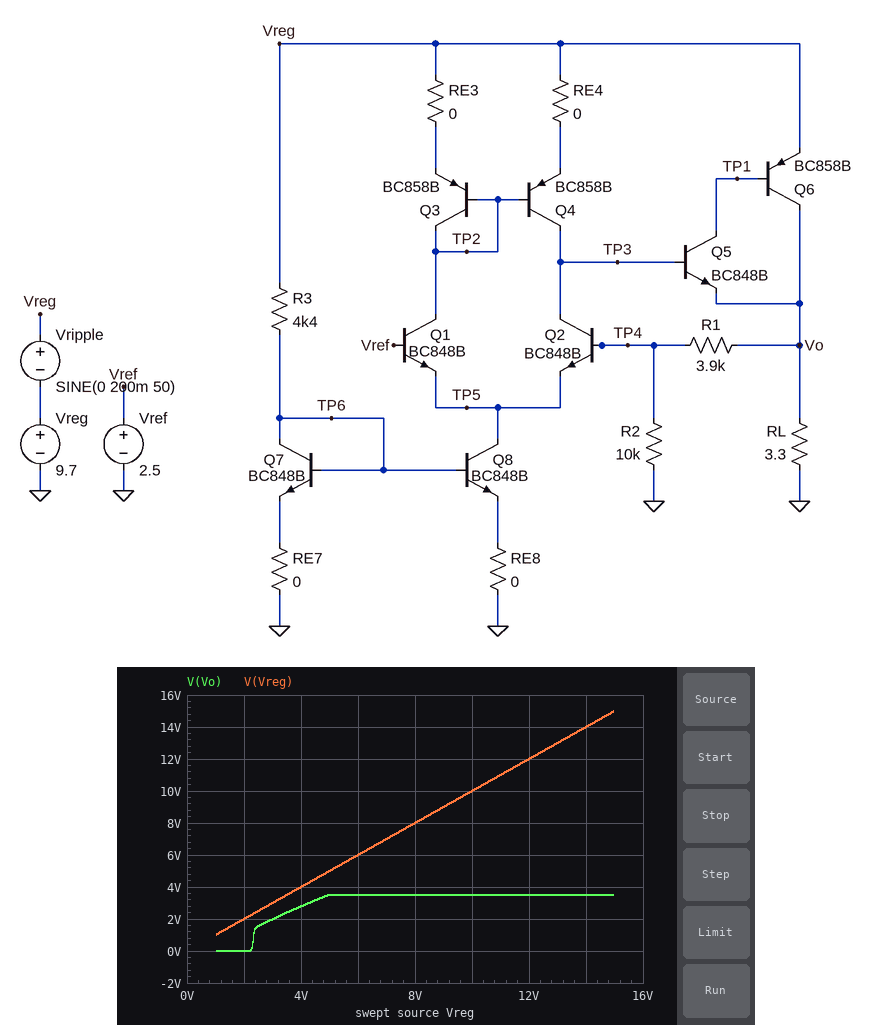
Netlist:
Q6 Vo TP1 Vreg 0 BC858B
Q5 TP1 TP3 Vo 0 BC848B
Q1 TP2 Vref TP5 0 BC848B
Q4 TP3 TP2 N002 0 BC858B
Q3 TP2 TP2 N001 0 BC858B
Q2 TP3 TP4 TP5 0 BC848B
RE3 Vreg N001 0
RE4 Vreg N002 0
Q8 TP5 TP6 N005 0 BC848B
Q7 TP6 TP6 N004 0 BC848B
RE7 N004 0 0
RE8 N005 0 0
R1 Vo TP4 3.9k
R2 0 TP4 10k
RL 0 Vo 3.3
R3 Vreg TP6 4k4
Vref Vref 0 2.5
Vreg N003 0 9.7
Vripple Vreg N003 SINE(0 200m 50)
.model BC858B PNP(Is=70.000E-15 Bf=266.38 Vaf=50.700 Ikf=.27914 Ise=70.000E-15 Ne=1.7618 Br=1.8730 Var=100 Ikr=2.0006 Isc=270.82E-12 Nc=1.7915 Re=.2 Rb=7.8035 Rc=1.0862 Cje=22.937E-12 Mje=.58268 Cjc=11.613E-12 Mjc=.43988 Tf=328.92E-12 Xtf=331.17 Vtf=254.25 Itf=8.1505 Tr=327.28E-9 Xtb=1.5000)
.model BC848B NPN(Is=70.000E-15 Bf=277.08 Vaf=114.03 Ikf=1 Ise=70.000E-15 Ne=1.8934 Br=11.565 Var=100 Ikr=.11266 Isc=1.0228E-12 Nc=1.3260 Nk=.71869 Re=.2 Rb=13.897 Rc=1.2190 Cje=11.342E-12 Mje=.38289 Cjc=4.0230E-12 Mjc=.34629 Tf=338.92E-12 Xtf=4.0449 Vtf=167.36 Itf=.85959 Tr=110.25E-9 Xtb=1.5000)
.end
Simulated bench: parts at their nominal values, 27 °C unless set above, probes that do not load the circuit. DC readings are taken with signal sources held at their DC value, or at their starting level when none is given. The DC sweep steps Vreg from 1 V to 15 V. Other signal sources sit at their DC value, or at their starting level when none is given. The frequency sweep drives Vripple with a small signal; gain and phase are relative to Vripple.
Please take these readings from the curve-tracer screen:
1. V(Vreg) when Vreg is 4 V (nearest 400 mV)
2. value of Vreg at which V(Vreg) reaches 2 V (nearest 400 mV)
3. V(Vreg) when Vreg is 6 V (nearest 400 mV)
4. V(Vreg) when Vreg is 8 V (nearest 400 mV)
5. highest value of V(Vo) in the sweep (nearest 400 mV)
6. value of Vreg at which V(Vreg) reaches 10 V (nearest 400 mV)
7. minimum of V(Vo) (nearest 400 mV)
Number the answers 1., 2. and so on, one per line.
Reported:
1. 4.0 V
2. 2.0 V
3. 6.0 V
4. 8.0 V
5. 3.6 V
6. 10.0 V
7. 0 V
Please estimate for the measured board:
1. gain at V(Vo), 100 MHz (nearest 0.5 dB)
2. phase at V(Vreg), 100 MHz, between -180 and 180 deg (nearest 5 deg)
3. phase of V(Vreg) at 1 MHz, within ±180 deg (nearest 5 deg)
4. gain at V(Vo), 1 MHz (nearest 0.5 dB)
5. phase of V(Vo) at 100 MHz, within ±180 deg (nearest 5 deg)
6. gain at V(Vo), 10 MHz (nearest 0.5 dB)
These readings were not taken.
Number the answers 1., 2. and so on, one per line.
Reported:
1. -19.5 dB
2. 0 deg
3. 0 deg
4. -42.5 dB
5. 0 deg
6. -16.0 dB
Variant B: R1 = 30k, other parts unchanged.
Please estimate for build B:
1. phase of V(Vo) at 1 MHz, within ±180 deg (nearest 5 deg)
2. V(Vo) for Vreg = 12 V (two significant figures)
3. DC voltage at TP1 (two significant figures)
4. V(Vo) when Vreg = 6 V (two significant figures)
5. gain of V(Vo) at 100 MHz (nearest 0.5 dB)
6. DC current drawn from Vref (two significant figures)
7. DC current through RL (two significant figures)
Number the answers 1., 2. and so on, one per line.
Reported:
1. 0 deg
2. 8.7 V
3. 7.3 V
4. 4.3 V
5. -2.5 dB
6. 7.1 µA
7. 2.1 A
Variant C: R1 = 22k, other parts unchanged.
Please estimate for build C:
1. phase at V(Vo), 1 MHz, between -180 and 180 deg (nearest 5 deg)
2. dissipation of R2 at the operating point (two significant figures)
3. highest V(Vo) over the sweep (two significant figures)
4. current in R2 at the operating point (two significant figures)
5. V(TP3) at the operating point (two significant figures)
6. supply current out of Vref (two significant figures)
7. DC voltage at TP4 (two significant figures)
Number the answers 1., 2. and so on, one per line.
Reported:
1. 0 deg
2. 480 µW
3. 8.1 V
4. 220 µA
5. 7.8 V
6. 7.1 µA
7. 2.2 V
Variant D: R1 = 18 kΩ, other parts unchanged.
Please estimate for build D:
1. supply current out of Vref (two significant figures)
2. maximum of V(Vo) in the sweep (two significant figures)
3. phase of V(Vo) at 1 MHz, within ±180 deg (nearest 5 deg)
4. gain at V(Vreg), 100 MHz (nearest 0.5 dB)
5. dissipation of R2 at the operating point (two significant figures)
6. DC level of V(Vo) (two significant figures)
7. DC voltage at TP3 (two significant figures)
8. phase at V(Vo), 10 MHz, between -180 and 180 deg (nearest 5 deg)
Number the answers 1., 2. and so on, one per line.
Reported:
1. 4.7 µA
2. 7.1 V
3. 5 deg
4. 0 dB
5. 620 µW
6. 7.0 V
7. 7.8 V
8. 0 deg
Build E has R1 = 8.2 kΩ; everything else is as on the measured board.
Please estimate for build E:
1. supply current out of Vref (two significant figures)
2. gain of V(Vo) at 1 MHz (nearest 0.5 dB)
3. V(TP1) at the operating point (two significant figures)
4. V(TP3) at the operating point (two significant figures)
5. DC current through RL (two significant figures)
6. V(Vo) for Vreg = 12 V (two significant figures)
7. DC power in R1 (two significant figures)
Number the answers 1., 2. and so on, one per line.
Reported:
1. 3.6 µA
2. -36.5 dB
3. 8.4 V
4. 5.3 V
5. 1.4 A
6. 4.6 V
7. 530 µW
